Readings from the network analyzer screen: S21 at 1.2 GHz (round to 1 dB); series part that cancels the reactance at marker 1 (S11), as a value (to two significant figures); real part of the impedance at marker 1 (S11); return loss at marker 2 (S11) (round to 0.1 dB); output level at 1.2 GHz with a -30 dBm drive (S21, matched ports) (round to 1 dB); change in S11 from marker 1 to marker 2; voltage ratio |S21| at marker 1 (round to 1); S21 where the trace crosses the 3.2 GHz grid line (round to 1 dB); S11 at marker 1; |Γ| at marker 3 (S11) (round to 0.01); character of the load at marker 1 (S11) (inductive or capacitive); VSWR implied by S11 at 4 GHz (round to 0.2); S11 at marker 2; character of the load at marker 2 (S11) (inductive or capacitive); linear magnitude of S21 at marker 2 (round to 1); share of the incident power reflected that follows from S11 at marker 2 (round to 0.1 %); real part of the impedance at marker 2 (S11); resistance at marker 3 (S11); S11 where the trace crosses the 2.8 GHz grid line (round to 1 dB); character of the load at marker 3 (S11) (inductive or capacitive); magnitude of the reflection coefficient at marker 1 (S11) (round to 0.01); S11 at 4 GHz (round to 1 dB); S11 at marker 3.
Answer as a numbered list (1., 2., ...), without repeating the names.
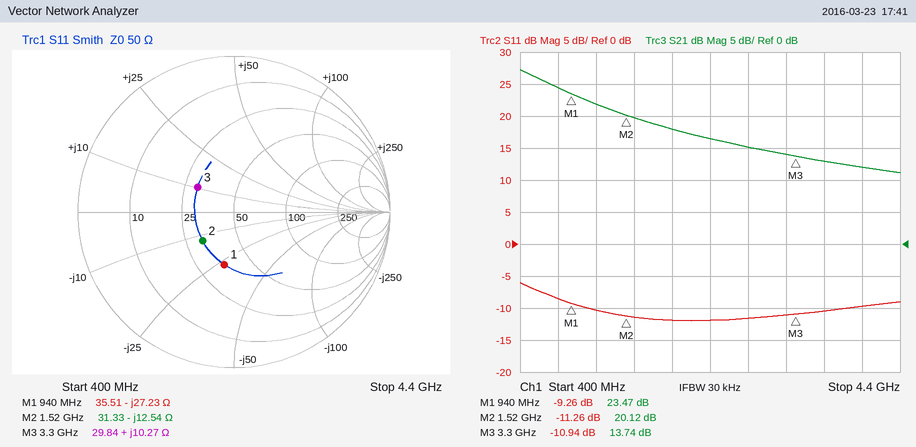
1. 22 dB
2. 4.6 nH
3. 35.51 Ω
4. 11.3 dB
5. -8 dBm
6. -2.00 dB
7. 15
8. 14 dB
9. -9.26 dB
10. 0.28
11. capacitive
12. 2.0
13. -11.26 dB
14. capacitive
15. 10
16. 7.5 %
17. 31.33 Ω
18. 29.84 Ω
19. -12 dB
20. inductive
21. 0.34
22. -10 dB
23. -10.94 dB
